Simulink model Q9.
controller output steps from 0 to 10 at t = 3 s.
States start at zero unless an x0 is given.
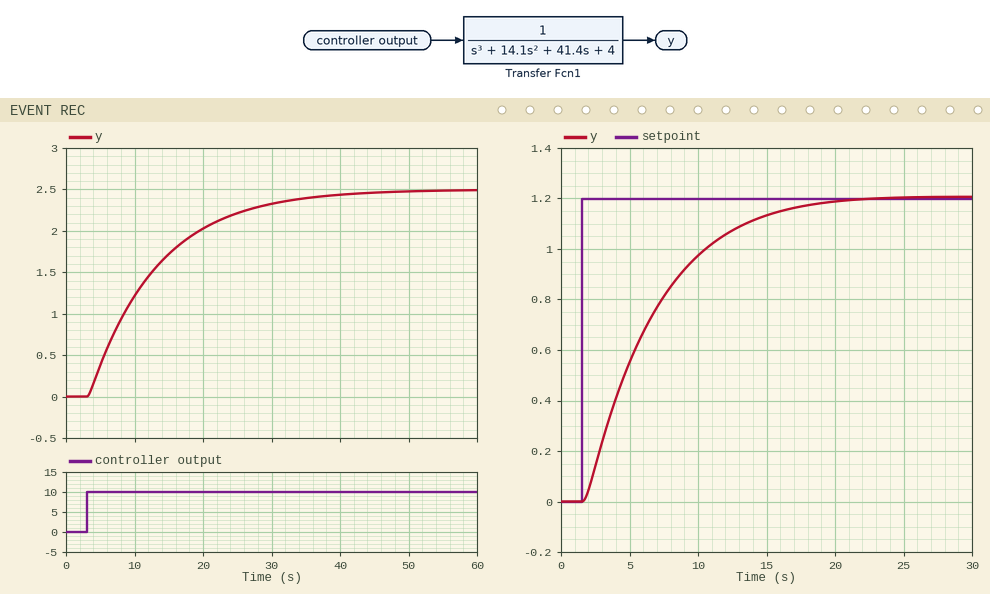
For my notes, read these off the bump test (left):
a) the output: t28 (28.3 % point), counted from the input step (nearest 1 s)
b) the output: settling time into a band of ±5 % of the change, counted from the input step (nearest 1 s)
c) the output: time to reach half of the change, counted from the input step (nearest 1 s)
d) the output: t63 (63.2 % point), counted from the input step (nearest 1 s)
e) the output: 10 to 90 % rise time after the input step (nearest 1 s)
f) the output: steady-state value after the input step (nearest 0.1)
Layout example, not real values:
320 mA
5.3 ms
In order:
4 s
30 s
7 s
10 s
22 s
2.5
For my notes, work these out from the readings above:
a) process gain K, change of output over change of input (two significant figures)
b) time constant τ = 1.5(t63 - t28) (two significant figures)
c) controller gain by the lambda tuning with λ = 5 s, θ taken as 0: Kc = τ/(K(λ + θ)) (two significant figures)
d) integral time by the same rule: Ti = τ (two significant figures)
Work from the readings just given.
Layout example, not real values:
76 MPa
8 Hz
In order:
0.25
9.0 s
7.2
9.0 s
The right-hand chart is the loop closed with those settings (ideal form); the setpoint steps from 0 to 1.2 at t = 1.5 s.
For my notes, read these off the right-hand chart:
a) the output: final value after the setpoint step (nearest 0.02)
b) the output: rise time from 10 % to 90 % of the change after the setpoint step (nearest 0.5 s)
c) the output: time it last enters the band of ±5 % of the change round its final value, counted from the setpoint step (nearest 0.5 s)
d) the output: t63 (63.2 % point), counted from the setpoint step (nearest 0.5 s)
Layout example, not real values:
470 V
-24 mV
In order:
1.20
10.5 s
14.0 s
5.5 s
